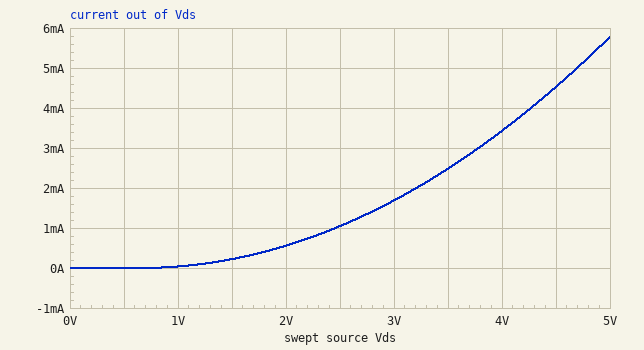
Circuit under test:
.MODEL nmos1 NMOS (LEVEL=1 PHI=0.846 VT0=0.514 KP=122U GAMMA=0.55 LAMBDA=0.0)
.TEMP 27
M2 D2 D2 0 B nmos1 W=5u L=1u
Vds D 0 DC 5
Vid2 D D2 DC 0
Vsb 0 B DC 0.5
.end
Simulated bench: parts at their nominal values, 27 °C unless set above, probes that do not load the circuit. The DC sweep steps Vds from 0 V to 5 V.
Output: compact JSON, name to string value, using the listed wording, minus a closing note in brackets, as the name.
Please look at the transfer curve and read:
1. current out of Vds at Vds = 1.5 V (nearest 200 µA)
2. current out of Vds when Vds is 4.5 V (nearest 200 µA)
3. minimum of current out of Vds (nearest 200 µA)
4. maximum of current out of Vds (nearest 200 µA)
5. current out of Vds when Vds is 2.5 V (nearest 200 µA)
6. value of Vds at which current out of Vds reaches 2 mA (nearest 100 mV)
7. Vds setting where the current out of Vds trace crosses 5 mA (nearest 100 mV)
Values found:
{"current out of Vds at Vds = 1.5 V": "200 µA", "current out of Vds when Vds is 4.5 V": "4.6 mA", "minimum of current out of Vds": "0 A", "maximum of current out of Vds": "5.8 mA", "current out of Vds when Vds is 2.5 V": "1.0 mA", "value of Vds at which current out of Vds reaches 2 mA": "3.2 V", "Vds setting where the current out of Vds trace crosses 5 mA": "4.7 V"}
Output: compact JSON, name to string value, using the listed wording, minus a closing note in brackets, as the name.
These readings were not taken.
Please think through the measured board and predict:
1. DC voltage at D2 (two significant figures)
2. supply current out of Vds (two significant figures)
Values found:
{"DC voltage at D2": "5.0 V", "supply current out of Vds": "5.8 mA"}
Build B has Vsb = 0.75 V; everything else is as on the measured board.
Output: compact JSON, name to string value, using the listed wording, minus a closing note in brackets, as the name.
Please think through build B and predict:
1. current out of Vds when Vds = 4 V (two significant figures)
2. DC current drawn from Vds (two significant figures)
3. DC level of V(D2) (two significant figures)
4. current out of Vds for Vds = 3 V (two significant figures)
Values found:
{"current out of Vds when Vds = 4 V": "3.3 mA", "DC current drawn from Vds": "5.6 mA", "DC level of V(D2)": "5.0 V", "current out of Vds for Vds = 3 V": "1.6 mA"}
